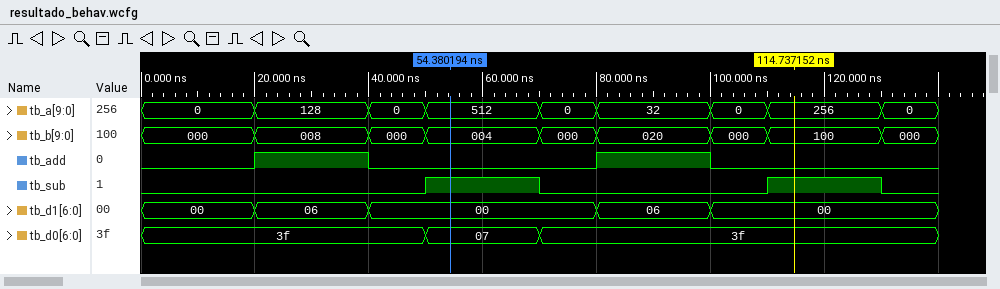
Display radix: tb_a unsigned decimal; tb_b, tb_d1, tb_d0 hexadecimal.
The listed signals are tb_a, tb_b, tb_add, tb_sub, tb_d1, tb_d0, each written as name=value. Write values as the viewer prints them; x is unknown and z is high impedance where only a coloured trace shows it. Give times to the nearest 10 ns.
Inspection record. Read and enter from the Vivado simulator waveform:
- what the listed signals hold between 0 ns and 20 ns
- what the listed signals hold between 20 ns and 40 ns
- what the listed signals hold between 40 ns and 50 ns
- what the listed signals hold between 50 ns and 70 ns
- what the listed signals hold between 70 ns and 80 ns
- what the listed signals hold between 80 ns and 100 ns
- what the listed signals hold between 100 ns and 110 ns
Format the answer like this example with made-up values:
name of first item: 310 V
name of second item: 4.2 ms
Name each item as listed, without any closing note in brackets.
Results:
what the listed signals hold between 0 ns and 20 ns: tb_a=0, tb_b=000, tb_add=0, tb_sub=0, tb_d1=00, tb_d0=3f
what the listed signals hold between 20 ns and 40 ns: tb_a=128, tb_b=008, tb_add=1, tb_sub=0, tb_d1=06, tb_d0=3f
what the listed signals hold between 40 ns and 50 ns: tb_a=0, tb_b=000, tb_add=0, tb_sub=0, tb_d1=00, tb_d0=3f
what the listed signals hold between 50 ns and 70 ns: tb_a=512, tb_b=004, tb_add=0, tb_sub=1, tb_d1=00, tb_d0=07
what the listed signals hold between 70 ns and 80 ns: tb_a=0, tb_b=000, tb_add=0, tb_sub=0, tb_d1=00, tb_d0=3f
what the listed signals hold between 80 ns and 100 ns: tb_a=32, tb_b=020, tb_add=1, tb_sub=0, tb_d1=06, tb_d0=3f
what the listed signals hold between 100 ns and 110 ns: tb_a=0, tb_b=000, tb_add=0, tb_sub=0, tb_d1=00, tb_d0=3f
